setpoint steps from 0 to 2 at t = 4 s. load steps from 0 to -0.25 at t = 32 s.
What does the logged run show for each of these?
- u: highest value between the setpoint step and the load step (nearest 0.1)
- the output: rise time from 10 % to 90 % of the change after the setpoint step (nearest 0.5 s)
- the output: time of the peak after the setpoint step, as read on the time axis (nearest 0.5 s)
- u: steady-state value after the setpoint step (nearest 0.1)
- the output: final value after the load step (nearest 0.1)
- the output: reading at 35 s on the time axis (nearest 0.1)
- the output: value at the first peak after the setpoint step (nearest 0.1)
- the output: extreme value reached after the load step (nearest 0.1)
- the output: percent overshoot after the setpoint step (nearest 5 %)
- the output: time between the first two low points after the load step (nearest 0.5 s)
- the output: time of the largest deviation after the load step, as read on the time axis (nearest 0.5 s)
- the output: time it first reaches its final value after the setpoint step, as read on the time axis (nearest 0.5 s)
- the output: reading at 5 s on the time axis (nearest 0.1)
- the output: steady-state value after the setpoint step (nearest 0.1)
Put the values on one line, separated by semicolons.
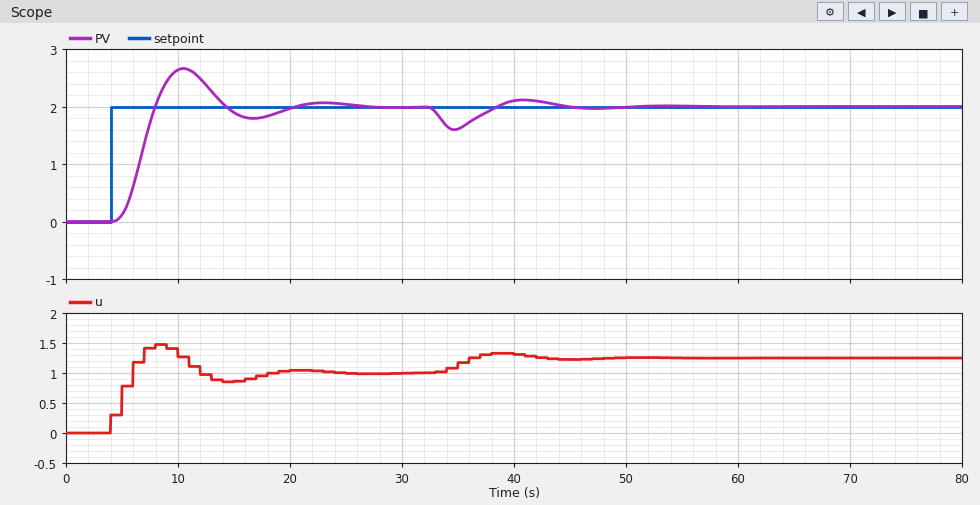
1.5; 2.5 s; 10.5 s; 1.0; 2.0; 1.6; 2.7; 1.6; 35 %; 12.5 s; 34.5 s; 8.0 s; 0.1; 2.0
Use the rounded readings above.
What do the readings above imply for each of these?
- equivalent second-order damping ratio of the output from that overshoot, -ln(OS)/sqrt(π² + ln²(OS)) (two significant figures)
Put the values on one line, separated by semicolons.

0.32
